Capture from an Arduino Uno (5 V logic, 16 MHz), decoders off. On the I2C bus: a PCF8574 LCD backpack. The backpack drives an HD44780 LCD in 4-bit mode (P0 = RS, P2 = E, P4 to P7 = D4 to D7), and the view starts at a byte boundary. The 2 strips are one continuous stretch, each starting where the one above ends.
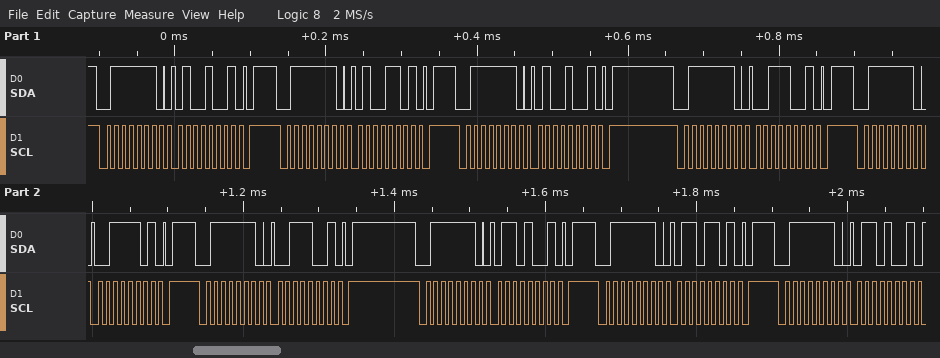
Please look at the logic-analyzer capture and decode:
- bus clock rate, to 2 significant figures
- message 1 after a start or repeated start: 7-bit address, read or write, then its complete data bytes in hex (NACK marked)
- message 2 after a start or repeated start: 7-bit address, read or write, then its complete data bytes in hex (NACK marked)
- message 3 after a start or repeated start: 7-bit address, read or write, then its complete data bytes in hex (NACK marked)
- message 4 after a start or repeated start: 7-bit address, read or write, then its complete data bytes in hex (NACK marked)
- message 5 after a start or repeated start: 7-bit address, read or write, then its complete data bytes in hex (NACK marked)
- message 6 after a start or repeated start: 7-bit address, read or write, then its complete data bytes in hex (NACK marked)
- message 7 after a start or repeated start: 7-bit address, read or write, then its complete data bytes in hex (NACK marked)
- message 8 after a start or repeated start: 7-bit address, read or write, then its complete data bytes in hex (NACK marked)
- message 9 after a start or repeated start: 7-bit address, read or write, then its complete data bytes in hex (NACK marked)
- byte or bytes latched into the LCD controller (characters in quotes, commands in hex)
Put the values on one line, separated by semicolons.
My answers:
100 kHz; 0x3F write: 49; 0x3F write: 4D; 0x3F write: 49; 0x3F write: 39; 0x3F write: 3D; 0x3F write: 39; 0x3F write: 69; 0x3F write: 6D; 0x3F write: 69; 'C'
